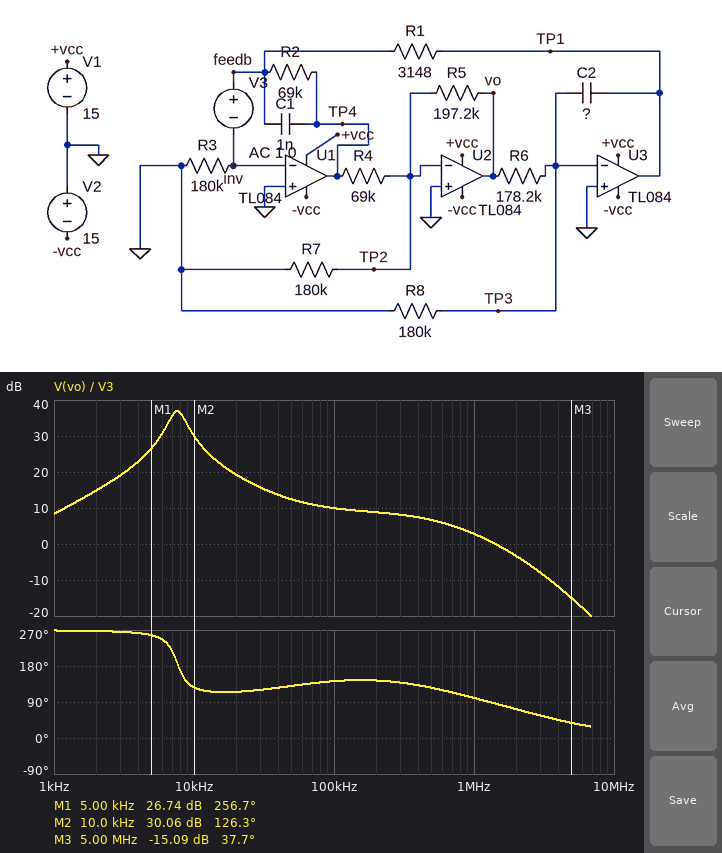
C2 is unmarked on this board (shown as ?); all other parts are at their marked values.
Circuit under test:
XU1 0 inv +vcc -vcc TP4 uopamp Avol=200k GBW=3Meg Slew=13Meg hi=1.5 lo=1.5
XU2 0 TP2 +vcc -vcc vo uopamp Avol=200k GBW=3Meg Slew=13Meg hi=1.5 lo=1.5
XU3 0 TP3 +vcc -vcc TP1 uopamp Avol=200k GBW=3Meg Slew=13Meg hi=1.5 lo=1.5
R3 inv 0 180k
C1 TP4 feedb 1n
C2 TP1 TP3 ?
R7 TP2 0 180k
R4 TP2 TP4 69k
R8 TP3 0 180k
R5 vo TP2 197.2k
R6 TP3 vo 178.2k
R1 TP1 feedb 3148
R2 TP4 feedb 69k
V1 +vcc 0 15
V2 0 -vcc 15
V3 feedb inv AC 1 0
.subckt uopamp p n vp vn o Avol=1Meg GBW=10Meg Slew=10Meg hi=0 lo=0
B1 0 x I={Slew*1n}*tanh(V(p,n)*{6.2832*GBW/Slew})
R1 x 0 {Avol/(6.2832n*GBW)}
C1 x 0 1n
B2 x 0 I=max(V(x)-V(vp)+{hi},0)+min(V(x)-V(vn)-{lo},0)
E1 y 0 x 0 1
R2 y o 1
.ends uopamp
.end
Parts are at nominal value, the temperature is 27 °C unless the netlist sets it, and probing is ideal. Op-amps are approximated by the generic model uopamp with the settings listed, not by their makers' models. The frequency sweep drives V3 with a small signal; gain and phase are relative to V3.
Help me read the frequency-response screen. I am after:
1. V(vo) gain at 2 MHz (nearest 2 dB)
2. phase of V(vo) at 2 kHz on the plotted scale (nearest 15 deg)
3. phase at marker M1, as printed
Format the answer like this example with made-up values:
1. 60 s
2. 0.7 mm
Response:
1. -4 dB
2. 270 deg
3. 256.7 deg
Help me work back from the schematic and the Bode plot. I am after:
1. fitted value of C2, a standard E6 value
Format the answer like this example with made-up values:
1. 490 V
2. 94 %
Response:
1. 2.2 nF
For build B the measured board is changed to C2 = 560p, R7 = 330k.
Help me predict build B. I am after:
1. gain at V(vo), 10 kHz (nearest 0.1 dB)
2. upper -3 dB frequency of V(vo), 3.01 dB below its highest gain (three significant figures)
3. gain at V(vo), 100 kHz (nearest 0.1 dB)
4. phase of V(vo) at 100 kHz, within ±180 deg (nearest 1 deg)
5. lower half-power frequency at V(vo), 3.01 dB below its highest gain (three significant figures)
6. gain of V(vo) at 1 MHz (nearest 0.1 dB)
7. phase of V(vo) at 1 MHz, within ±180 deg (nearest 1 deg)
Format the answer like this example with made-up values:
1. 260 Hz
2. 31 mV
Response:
1. 21.5 dB
2. 16.0 kHz
3. 10.1 dB
4. 143 deg
5. 14.2 kHz
6. 3.5 dB
7. 103 deg
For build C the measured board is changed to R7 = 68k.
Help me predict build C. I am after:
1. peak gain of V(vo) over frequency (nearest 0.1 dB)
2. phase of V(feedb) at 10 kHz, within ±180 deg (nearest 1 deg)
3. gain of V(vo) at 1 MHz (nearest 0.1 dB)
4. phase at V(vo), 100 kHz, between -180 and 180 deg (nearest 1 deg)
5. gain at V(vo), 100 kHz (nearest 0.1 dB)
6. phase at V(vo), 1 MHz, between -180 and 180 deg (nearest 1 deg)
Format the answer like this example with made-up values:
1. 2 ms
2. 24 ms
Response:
1. 37.1 dB
2. -1 deg
3. 0.7 dB
4. 139 deg
5. 9.9 dB
6. 93 deg
